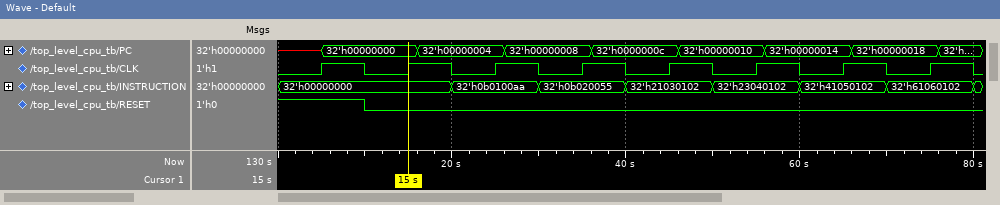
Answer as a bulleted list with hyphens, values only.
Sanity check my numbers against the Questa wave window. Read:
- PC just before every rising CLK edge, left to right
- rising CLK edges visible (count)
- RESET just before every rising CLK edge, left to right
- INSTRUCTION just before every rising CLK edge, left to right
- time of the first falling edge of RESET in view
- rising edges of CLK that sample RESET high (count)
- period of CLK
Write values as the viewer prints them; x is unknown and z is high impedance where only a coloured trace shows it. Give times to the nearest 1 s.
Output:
- x, 32'h00000000, 32'h00000004, 32'h00000008, 32'h0000000c, 32'h00000010, 32'h00000014, 32'h00000018
- 8
- 1 0 0 0 0 0 0 0
- 32'h00000000, 32'h00000000, 32'h0b0100aa, 32'h0b020055, 32'h21030102, 32'h23040102, 32'h41050102, 32'h61060102
- 10 s
- 1
- 10 s
